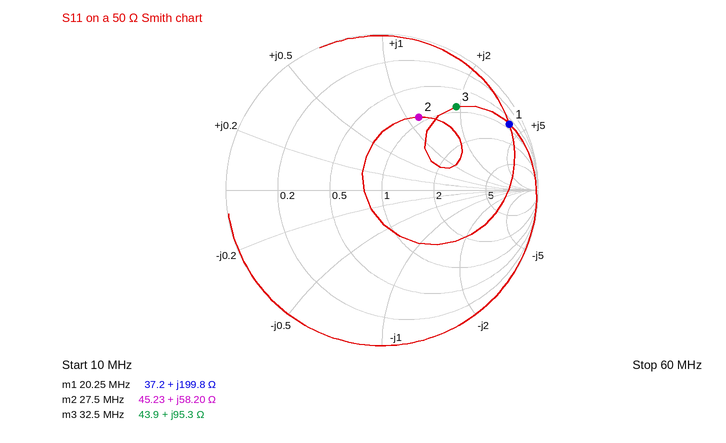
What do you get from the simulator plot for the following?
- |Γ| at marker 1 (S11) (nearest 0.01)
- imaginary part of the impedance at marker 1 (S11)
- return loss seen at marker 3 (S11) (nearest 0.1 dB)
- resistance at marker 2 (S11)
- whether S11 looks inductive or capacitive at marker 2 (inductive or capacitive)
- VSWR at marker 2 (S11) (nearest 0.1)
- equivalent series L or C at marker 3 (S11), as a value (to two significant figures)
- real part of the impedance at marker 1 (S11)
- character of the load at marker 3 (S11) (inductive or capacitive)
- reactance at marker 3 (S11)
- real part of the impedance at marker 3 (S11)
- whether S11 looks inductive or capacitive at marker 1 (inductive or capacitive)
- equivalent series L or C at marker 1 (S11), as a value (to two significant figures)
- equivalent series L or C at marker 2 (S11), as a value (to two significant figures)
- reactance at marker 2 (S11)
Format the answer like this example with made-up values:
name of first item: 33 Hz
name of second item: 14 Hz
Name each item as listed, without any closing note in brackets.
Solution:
|Γ| at marker 1 (S11): 0.92
imaginary part of the impedance at marker 1: +199.8 Ω
return loss seen at marker 3 (S11): 2.9 dB
resistance at marker 2: 45.23 Ω
whether S11 looks inductive or capacitive at marker 2: inductive
VSWR at marker 2 (S11): 3.2
equivalent series L or C at marker 3 (S11), as a value: 470 nH
real part of the impedance at marker 1: 37.2 Ω
character of the load at marker 3 (S11): inductive
reactance at marker 3: +95.3 Ω
real part of the impedance at marker 3: 43.9 Ω
whether S11 looks inductive or capacitive at marker 1: inductive
equivalent series L or C at marker 1 (S11), as a value: 1.6 µH
equivalent series L or C at marker 2 (S11), as a value: 340 nH
reactance at marker 2: +58.20 Ω
